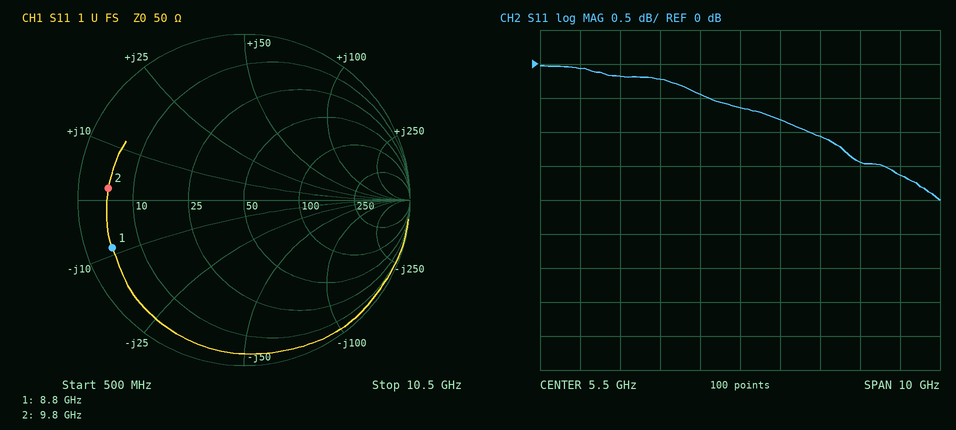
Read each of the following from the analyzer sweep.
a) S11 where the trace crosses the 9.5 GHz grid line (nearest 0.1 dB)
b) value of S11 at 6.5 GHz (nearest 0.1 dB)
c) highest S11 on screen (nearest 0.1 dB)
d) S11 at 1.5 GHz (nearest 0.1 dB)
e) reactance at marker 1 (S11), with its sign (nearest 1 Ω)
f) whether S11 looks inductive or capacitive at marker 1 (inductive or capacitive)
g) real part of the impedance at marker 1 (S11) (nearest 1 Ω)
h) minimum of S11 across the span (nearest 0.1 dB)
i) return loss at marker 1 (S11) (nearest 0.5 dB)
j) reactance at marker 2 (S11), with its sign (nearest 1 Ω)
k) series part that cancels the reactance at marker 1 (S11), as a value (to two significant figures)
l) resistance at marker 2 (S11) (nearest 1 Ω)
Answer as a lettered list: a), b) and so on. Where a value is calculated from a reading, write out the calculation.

a) -1.6 dB
b) -0.8 dB
c) 0.0 dB
d) -0.1 dB
e) -9 Ω
f) capacitive
g) 4 Ω
h) -2.0 dB
i) 1.5 dB
j) +2 Ω
k) L = 9 Ω/(2π × 8.8 GHz) ≈ 163 pH, so 160 pH to two significant figures
l) 5 Ω
